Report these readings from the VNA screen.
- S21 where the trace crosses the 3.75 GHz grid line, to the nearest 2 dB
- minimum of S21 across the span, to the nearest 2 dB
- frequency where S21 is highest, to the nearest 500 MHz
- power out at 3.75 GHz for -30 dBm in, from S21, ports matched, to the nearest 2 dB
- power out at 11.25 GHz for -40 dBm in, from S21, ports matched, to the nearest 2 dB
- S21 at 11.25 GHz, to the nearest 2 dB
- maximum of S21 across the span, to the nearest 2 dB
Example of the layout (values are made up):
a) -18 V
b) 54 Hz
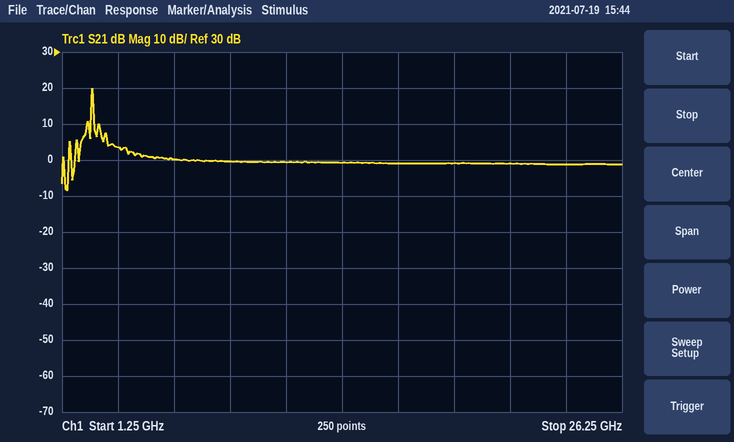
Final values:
a) 4 dB
b) -8 dB
c) 2.5 GHz
d) -26 dBm
e) -40 dBm
f) 0 dB
g) 20 dB
